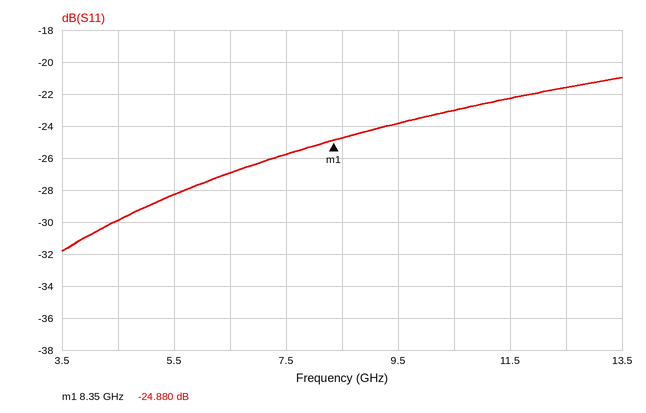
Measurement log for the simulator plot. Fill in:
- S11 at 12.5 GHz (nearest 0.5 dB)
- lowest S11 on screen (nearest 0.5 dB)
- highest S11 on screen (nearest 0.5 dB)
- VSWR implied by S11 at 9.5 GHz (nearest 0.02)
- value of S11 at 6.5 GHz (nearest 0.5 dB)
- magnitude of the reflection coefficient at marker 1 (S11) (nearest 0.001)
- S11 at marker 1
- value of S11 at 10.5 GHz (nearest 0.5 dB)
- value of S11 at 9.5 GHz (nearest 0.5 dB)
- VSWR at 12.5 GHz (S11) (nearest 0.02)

-21.5 dB
-32.0 dB
-21.0 dB
1.14
-27.0 dB
0.057
-24.880 dB
-23.0 dB
-24.0 dB
1.18
